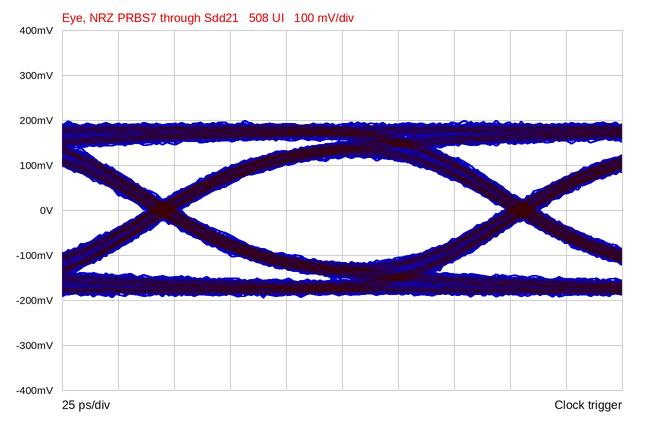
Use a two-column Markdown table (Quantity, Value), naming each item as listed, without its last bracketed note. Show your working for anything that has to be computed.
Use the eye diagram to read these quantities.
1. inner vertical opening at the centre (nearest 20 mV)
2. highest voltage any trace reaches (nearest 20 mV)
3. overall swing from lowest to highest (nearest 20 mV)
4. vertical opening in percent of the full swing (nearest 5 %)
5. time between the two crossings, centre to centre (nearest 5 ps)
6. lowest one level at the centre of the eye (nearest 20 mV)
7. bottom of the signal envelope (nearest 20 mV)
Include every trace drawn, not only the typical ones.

| Quantity | Value |
|---|---|
| inner vertical opening at the centre | 240 mV |
| highest voltage any trace reaches | 200 mV |
| overall swing from lowest to highest | 400 mV |
| vertical opening in percent of the full swing | 240 mV / 400 mV ≈ 60 % |
| time between the two crossings, centre to centre | 160 ps |
| lowest one level at the centre of the eye | 120 mV |
| bottom of the signal envelope | -200 mV |
